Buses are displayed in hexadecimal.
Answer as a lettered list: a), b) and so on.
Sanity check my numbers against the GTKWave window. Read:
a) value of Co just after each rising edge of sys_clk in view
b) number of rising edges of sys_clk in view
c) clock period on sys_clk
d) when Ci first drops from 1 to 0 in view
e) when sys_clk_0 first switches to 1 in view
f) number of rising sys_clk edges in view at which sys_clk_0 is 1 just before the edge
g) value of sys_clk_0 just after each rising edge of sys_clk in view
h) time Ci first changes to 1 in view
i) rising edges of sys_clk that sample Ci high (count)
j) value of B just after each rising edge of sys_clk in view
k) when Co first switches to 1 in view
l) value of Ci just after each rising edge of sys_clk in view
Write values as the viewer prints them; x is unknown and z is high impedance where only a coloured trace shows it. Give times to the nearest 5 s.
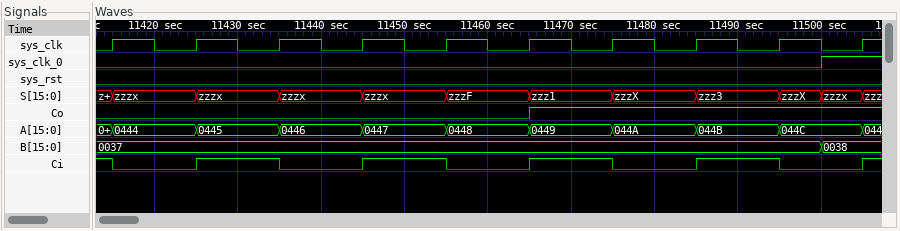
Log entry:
a) 0 0 0 0 0 1 1 1 1 1
b) 10
c) 10 s
d) 11415 s
e) 11500 s
f) 1
g) 0 0 0 0 0 0 0 0 0 1
h) 11425 s
i) 5
j) 0037, 0037, 0037, 0037, 0037, 0037, 0037, 0037, 0037, 0038
k) 11465 s
l) 0 1 0 1 0 1 0 1 0 1
